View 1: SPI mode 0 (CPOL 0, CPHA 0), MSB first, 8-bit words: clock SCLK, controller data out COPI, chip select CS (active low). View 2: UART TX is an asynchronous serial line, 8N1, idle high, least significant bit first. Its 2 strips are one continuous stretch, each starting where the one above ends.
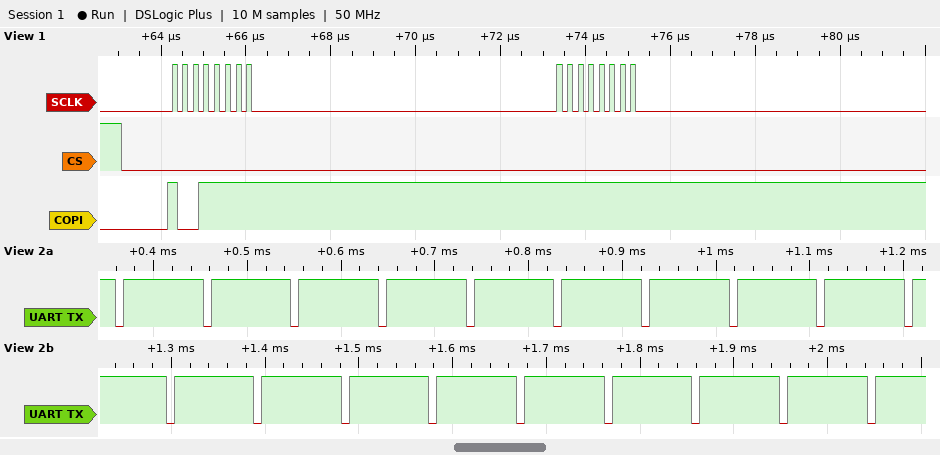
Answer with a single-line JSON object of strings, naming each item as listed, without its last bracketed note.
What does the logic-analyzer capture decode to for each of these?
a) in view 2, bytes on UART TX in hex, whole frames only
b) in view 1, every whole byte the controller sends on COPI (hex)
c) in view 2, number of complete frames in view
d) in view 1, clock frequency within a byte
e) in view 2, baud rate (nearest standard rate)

{"in view 2, bytes on UART TX in hex, whole frames only": "FF FF FF FF FF FF FF FF FF FF FF FF FF FF FF FF FF FF", "in view 1, every whole byte the controller sends on COPI": "9F FF", "in view 2, number of complete frames in view": "18", "in view 1, clock frequency within a byte": "4 MHz", "in view 2, baud rate": "115200 baud"}
